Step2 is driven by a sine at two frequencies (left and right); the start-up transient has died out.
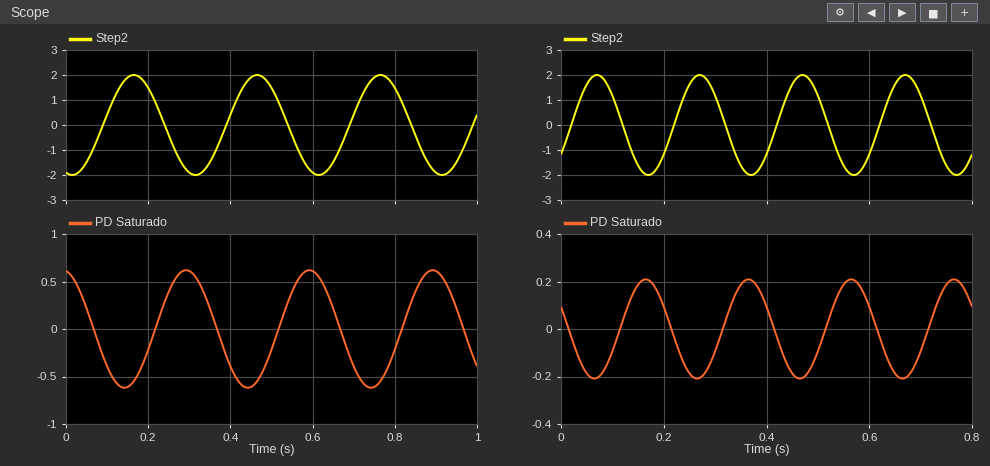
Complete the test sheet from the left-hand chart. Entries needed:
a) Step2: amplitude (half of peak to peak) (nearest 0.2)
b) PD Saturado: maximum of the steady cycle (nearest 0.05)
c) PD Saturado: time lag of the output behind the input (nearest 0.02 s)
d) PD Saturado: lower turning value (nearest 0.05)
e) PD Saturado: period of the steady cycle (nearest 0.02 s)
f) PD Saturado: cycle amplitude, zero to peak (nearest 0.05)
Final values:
2.0
0.60
0.12 s
-0.60
0.30 s
0.60
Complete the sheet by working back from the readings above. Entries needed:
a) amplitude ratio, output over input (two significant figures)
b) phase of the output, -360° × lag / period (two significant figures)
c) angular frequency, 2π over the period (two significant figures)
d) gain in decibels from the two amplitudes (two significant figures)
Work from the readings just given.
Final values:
0.30
-140°
21 rad/s
-10 dB
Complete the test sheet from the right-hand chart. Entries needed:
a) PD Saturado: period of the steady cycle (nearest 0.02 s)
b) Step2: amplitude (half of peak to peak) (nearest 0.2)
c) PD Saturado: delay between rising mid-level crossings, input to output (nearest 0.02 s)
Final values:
0.20 s
2.0
0.10 s
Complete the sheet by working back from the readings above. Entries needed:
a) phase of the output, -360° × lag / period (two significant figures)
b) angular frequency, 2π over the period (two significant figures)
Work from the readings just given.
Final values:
-180°
31 rad/s
